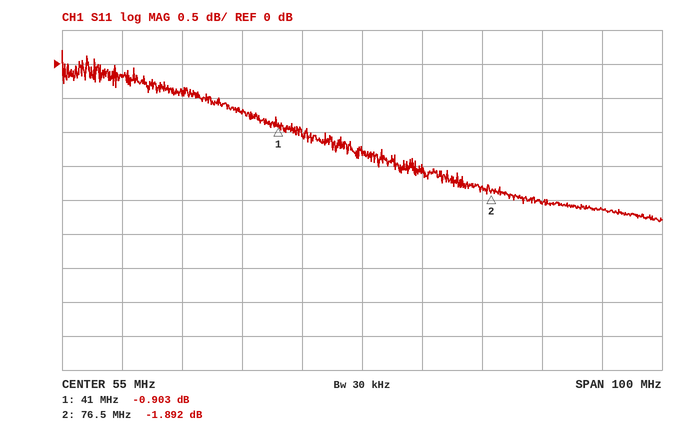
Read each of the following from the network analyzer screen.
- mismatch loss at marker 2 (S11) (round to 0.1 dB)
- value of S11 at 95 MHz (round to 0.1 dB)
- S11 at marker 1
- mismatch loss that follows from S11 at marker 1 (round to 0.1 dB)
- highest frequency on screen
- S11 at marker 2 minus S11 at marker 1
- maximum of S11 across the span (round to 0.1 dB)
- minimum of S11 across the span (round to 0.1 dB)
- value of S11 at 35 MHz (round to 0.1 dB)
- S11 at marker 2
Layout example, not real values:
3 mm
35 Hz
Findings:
4.5 dB
-2.1 dB
-0.903 dB
7.3 dB
105 MHz
-0.989 dB
0.2 dB
-2.3 dB
-0.7 dB
-1.892 dB
